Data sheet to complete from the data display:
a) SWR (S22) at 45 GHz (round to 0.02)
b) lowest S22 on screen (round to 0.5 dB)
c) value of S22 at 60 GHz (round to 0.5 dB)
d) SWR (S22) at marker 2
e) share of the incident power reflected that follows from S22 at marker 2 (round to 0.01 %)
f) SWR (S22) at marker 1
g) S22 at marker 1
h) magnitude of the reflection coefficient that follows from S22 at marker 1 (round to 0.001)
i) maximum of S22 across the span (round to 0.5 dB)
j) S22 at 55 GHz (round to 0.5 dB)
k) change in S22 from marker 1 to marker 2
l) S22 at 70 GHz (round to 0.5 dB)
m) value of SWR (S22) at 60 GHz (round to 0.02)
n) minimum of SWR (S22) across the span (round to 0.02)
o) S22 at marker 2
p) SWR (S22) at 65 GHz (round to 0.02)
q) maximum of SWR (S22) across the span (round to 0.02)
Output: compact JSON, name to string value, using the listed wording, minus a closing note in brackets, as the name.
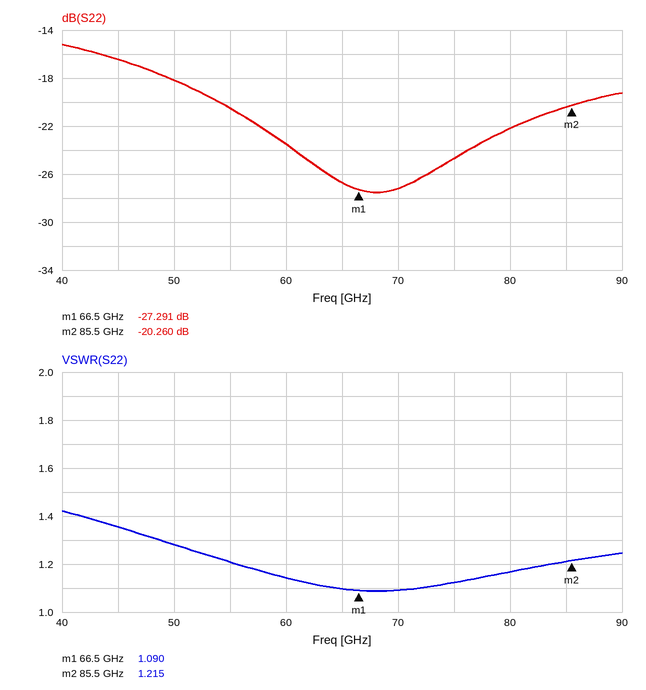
{"SWR (S22) at 45 GHz": "1.36", "lowest S22 on screen": "-27.5 dB", "value of S22 at 60 GHz": "-23.5 dB", "SWR (S22) at marker 2": "1.215", "share of the incident power reflected that follows from S22 at marker 2": "0.94 %", "SWR (S22) at marker 1": "1.090", "S22 at marker 1": "-27.291 dB", "magnitude of the reflection coefficient that follows from S22 at marker 1": "0.043", "maximum of S22 across the span": "-15.0 dB", "S22 at 55 GHz": "-20.5 dB", "change in S22 from marker 1 to marker 2": "7.031 dB", "S22 at 70 GHz": "-27.0 dB", "value of SWR (S22) at 60 GHz": "1.14", "minimum of SWR (S22) across the span": "1.08", "S22 at marker 2": "-20.260 dB", "SWR (S22) at 65 GHz": "1.10", "maximum of SWR (S22) across the span": "1.42"}
